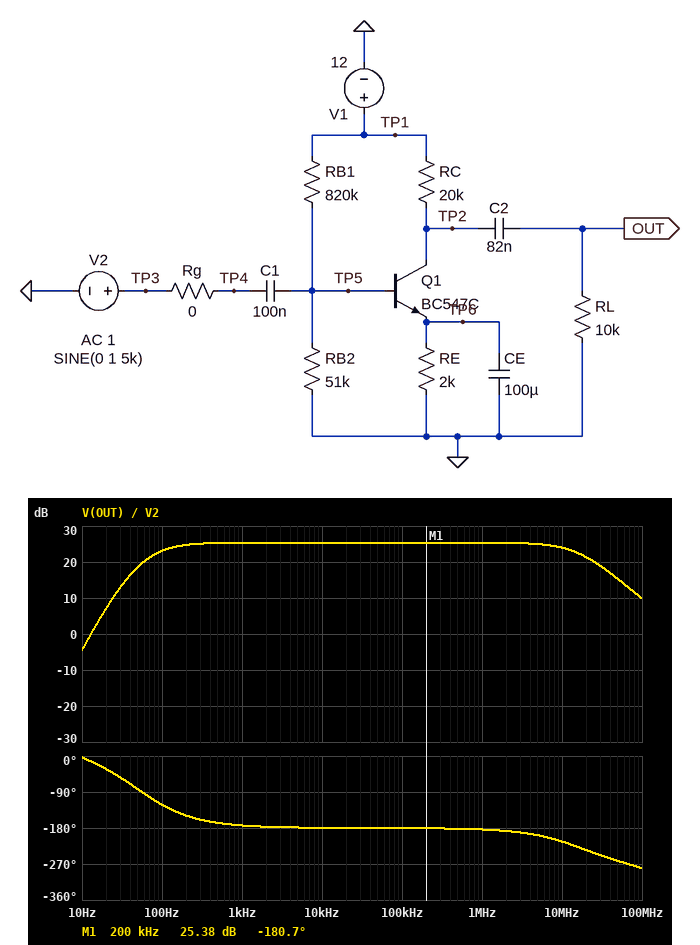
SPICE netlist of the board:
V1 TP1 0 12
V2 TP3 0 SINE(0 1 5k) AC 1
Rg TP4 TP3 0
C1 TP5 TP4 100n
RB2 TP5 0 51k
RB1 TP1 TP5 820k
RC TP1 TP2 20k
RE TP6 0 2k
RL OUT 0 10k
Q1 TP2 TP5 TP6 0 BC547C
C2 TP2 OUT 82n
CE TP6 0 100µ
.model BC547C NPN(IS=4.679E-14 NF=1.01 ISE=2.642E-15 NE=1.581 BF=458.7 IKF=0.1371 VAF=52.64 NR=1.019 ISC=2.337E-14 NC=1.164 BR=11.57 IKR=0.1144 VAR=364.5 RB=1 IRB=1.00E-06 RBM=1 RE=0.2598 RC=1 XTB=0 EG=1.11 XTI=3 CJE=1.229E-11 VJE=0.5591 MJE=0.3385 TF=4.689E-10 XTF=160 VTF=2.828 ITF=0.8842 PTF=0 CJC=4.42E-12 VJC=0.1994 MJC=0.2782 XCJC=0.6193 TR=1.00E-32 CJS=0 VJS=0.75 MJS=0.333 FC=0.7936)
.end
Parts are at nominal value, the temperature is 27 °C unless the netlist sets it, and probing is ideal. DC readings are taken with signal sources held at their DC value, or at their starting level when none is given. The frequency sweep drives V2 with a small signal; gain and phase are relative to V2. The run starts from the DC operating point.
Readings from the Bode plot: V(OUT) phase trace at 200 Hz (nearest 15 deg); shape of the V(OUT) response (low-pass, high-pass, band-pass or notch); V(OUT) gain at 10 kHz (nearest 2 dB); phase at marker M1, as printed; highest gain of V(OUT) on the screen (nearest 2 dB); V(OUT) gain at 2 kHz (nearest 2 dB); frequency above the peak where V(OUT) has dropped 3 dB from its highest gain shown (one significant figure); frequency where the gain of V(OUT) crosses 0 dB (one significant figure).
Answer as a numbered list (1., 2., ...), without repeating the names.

1. -150 deg
2. band-pass
3. 26 dB
4. -180.7 deg
5. 26 dB
6. 26 dB
7. 20 MHz
8. 10 Hz
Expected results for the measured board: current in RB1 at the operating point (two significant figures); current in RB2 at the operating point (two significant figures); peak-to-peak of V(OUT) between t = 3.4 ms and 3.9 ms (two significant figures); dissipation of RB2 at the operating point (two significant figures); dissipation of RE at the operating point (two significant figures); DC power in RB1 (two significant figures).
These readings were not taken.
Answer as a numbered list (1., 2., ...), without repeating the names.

1. 14 µA
2. 14 µA
3. 9.9 V
4. 9.5 µW
5. 11 µW
6. 160 µW
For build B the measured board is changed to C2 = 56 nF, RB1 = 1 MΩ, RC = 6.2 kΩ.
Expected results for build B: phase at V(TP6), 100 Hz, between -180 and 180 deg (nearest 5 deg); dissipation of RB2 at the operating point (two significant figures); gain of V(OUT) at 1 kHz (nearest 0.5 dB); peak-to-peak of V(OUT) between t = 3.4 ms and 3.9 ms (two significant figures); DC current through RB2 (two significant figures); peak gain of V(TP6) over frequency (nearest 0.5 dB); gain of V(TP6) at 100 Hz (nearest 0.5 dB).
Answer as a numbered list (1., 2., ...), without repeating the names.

1. -70 deg
2. 6.6 µW
3. 12.0 dB
4. 11 V
5. 11 µA
6. -27.0 dB
7. -36.0 dB
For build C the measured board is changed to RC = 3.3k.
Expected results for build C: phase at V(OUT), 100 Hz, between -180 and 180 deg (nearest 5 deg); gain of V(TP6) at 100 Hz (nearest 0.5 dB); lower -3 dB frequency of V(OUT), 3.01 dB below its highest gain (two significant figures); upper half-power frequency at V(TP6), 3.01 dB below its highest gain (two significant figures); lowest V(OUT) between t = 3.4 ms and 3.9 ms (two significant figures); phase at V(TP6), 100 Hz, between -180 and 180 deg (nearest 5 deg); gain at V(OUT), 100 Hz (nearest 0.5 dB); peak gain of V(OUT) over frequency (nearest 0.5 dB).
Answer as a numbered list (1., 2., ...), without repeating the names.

1. -100 deg
2. -27.5 dB
3. 160 Hz
4. 50 Hz
5. -10 V
6. -65 deg
7. 11.0 dB
8. 17.0 dB
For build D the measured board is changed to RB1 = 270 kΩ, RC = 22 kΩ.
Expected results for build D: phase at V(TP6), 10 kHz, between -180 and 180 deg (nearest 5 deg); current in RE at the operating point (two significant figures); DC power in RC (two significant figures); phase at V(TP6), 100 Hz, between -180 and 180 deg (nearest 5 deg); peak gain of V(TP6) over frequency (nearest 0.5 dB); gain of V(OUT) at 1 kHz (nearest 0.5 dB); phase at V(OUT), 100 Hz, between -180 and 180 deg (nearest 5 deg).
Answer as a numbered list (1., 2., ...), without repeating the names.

1. -70 deg
2. 500 µA
3. 5.4 mW
4. 5 deg
5. -56.0 dB
6. 8.0 dB
7. -30 deg
